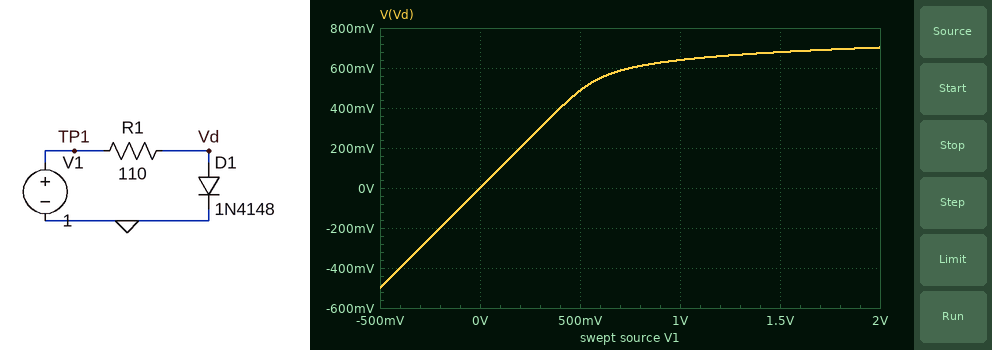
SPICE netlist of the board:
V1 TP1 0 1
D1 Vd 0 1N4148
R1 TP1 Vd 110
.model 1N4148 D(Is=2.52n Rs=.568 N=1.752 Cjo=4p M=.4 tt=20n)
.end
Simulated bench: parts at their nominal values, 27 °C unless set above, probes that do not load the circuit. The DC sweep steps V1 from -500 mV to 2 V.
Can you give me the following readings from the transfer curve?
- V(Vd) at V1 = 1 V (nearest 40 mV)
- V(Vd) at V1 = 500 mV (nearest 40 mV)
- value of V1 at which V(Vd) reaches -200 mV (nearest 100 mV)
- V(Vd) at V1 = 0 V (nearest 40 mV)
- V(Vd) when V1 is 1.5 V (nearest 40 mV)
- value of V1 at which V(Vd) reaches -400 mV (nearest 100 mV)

640 mV
480 mV
-200 mV
0 V
680 mV
-400 mV
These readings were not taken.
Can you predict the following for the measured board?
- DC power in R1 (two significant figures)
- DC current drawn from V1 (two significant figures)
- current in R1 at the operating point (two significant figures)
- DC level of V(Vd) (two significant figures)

1.2 mW
3.3 mA
3.3 mA
640 mV
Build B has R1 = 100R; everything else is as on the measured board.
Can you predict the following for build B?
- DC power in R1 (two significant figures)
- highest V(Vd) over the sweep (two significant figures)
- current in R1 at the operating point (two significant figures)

1.3 mW
710 mV
3.6 mA
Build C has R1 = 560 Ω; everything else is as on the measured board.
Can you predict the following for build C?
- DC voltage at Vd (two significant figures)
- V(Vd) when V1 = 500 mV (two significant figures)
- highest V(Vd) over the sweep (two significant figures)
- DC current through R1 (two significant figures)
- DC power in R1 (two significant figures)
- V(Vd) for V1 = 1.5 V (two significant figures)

570 mV
460 mV
630 mV
760 µA
330 µW
610 mV
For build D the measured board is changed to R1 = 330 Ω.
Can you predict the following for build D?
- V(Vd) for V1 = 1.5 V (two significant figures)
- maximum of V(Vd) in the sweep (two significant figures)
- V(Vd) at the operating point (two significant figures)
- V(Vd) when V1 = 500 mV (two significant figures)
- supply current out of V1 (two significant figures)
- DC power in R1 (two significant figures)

630 mV
650 mV
590 mV
470 mV
1.2 mA
500 µW
